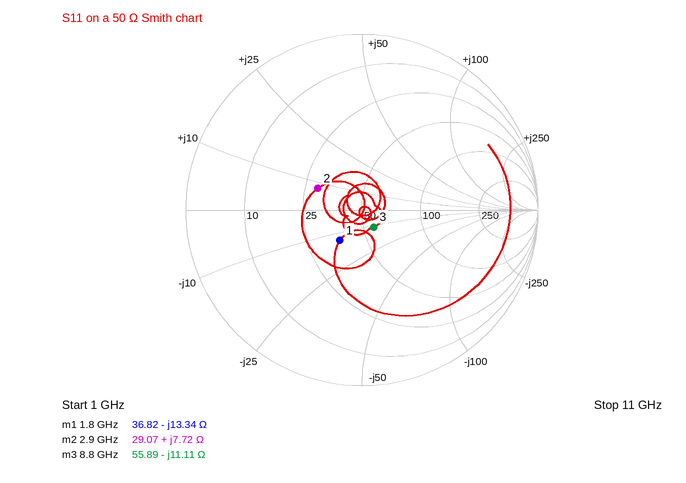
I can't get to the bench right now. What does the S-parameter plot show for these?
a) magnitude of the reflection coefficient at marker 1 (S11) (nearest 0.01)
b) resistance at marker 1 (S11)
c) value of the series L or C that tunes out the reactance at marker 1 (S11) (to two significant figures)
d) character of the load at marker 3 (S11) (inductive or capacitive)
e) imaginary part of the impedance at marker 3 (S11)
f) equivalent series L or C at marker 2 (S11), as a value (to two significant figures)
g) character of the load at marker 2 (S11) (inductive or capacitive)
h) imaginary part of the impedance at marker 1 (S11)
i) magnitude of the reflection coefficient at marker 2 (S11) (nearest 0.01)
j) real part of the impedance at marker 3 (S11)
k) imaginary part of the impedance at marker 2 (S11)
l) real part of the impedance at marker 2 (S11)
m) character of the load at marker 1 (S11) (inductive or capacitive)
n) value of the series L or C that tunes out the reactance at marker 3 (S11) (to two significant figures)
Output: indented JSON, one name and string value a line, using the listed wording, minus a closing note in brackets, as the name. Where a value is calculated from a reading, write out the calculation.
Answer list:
{
  "magnitude of the reflection coefficient at marker 1 (S11)": "0.21",
  "resistance at marker 1": "36.82 Ω",
  "value of the series L or C that tunes out the reactance at marker 1 (S11)": "L = 13.34 Ω/(2π × 1.8 GHz) ≈ 1.2 nH",
  "character of the load at marker 3 (S11)": "capacitive",
  "imaginary part of the impedance at marker 3": "-11.11 Ω",
  "equivalent series L or C at marker 2 (S11), as a value": "L = 7.72 Ω/(2π × 2.9 GHz) ≈ 424 pH, so 420 pH to two significant figures",
  "character of the load at marker 2 (S11)": "inductive",
  "imaginary part of the impedance at marker 1": "-13.34 Ω",
  "magnitude of the reflection coefficient at marker 2 (S11)": "0.28",
  "real part of the impedance at marker 3": "55.89 Ω",
  "imaginary part of the impedance at marker 2": "+7.72 Ω",
  "real part of the impedance at marker 2": "29.07 Ω",
  "character of the load at marker 1 (S11)": "capacitive",
  "value of the series L or C that tunes out the reactance at marker 3 (S11)": "L = 11.11 Ω/(2π × 8.8 GHz) ≈ 201 pH, so 200 pH to two significant figures"
}
